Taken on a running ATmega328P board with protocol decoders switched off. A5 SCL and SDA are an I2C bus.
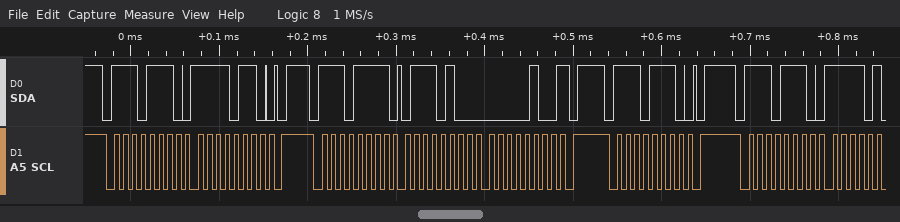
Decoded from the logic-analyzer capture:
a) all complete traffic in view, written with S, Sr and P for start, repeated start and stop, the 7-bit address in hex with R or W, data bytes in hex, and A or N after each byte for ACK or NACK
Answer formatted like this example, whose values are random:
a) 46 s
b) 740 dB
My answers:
a) S 77W A F6 A P S 77R A 74 A 04 N P S 77W A P S 77W A
